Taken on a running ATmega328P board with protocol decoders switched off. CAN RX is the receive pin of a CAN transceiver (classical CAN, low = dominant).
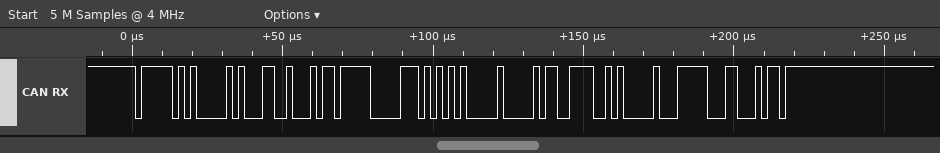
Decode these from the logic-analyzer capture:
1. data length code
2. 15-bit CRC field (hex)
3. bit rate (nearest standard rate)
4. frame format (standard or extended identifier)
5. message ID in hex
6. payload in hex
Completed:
8
0x7CC5
500 kbit/s
standard
0x7E8
C8 B7 C3 55 00 19 E5 00
